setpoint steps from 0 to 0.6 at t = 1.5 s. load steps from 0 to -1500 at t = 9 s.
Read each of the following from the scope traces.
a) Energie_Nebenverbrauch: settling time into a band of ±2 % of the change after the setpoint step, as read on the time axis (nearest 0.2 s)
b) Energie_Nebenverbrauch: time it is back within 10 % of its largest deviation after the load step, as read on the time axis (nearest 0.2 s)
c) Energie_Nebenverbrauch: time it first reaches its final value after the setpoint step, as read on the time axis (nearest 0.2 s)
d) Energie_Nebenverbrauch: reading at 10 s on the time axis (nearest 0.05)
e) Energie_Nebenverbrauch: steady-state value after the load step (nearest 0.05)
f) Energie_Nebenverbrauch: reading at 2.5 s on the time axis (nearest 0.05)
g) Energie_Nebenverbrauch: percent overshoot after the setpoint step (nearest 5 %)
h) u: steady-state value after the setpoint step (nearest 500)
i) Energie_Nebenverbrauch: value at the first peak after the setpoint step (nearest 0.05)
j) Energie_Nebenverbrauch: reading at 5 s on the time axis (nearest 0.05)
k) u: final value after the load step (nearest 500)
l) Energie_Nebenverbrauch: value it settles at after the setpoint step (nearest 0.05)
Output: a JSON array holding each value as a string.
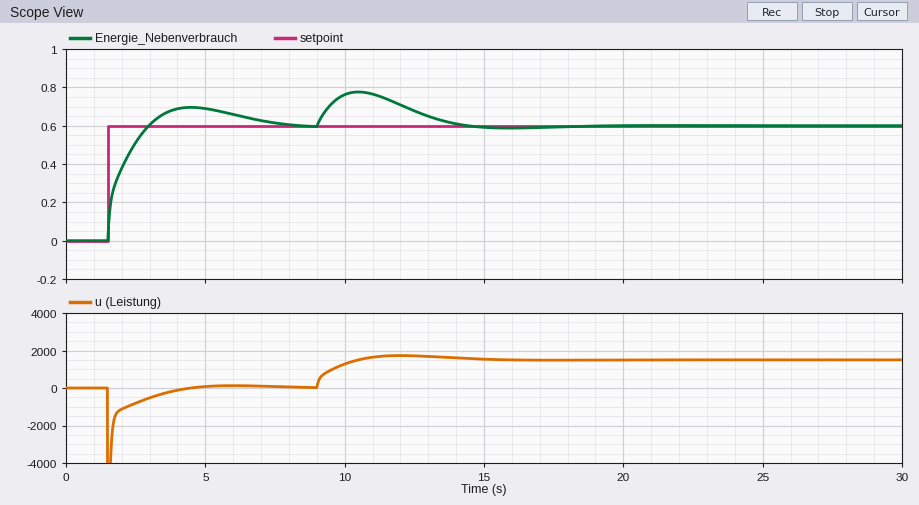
["7.6 s", "13.8 s", "3.0 s", "0.75", "0.60", "0.50", "15 %", "0", "0.70", "0.70", "1500", "0.60"]
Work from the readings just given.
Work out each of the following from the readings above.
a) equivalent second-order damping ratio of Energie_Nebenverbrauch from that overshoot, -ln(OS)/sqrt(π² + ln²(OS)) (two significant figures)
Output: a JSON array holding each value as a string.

["0.52"]
